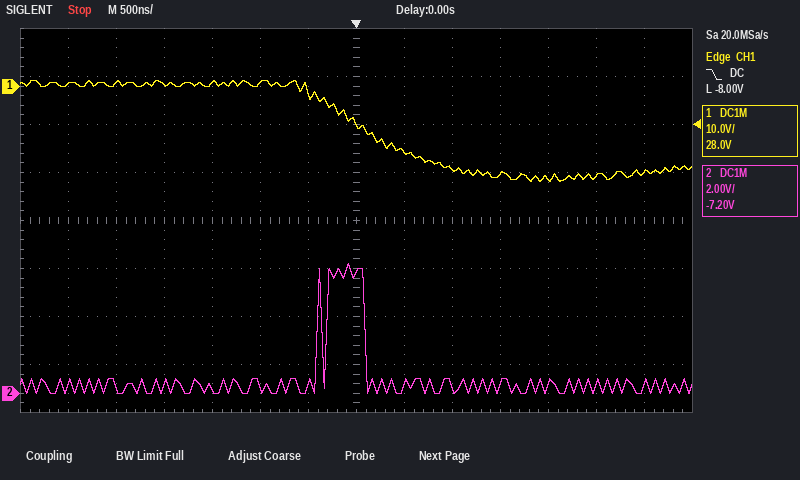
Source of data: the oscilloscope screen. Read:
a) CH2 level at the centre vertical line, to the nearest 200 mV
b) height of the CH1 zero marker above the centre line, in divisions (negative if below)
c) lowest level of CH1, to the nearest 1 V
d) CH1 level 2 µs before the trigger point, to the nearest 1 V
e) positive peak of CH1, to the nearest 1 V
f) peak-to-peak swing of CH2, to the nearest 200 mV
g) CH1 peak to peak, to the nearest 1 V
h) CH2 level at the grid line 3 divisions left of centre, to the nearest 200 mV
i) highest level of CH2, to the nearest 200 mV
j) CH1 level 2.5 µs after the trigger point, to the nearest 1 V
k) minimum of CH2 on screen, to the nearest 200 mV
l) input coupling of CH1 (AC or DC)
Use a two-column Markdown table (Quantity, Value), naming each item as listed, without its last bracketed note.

| Quantity | Value |
|---|---|
| CH2 level at the centre vertical line, to the nearest 200 mV | 5.0 V |
| height of the CH1 zero marker above the centre line, in divisions | +2.8 div |
| lowest level of CH1, to the nearest 1 V | -20 V |
| CH1 level 2 µs before the trigger point, to the nearest 1 V | 0 V |
| positive peak of CH1, to the nearest 1 V | 1 V |
| peak-to-peak swing of CH2, to the nearest 200 mV | 5.4 V |
| CH1 peak to peak, to the nearest 1 V | 21 V |
| CH2 level at the grid line 3 divisions left of centre, to the nearest 200 mV | 200 mV |
| highest level of CH2, to the nearest 200 mV | 5.4 V |
| CH1 level 2.5 µs after the trigger point, to the nearest 1 V | -19 V |
| minimum of CH2 on screen, to the nearest 200 mV | 0.0 V |
| input coupling of CH1 | DC |
